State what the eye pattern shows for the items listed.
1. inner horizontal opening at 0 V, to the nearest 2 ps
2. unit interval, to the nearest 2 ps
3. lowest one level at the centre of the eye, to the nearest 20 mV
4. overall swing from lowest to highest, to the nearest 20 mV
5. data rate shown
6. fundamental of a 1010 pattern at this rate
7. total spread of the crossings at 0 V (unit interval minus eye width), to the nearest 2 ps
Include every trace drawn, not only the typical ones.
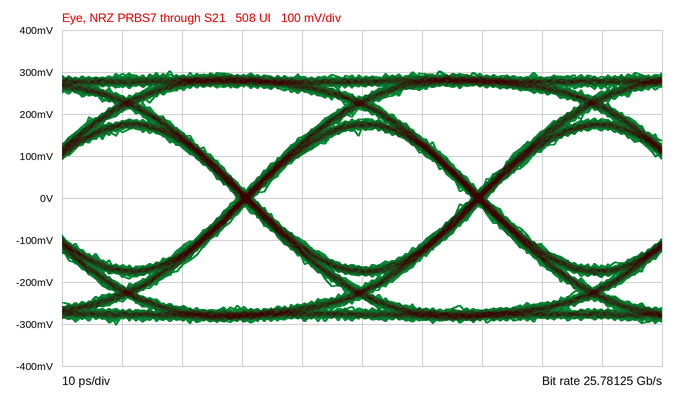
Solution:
36 ps
38 ps
160 mV
600 mV
25.78125 Gb/s
12.89062 GHz
2 ps
